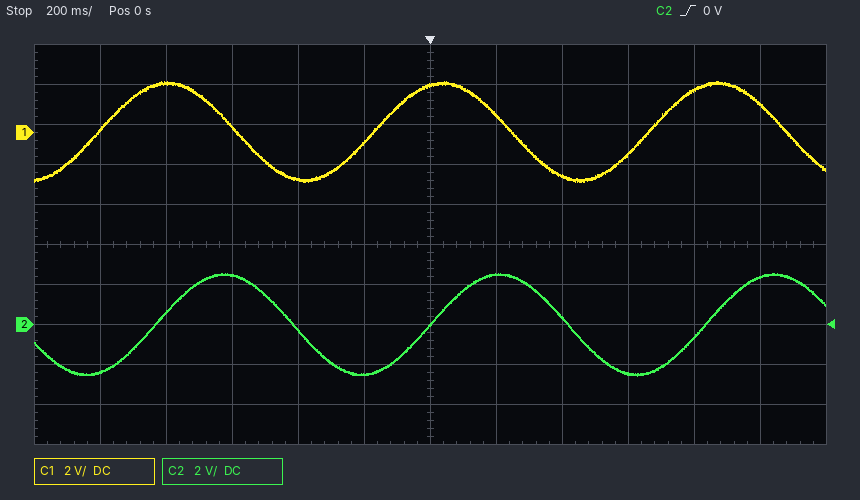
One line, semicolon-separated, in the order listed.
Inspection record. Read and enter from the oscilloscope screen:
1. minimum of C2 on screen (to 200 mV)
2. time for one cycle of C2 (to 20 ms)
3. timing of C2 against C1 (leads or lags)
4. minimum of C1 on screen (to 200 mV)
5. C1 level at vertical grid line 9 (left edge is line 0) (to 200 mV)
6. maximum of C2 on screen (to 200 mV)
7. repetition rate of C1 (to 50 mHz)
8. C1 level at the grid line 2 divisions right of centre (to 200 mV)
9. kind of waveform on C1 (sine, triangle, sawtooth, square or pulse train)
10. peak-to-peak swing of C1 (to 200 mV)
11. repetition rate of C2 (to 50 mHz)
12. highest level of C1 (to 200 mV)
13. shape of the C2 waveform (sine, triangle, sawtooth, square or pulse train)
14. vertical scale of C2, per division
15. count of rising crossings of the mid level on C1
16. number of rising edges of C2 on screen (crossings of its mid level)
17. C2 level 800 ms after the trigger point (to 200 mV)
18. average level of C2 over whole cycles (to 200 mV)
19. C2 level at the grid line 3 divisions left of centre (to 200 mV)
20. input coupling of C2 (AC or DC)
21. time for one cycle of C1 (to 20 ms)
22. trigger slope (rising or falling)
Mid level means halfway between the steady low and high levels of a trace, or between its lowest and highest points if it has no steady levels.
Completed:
-2.6 V; 840 ms; lags; -2.4 V; -1.0 V; 2.6 V; 1.20 Hz; -2.2 V; sine; 5.0 V; 1.20 Hz; 2.6 V; sine; 2 V; 3; 3; -600 mV; 0.0 V; 2.4 V; DC; 840 ms; rising
